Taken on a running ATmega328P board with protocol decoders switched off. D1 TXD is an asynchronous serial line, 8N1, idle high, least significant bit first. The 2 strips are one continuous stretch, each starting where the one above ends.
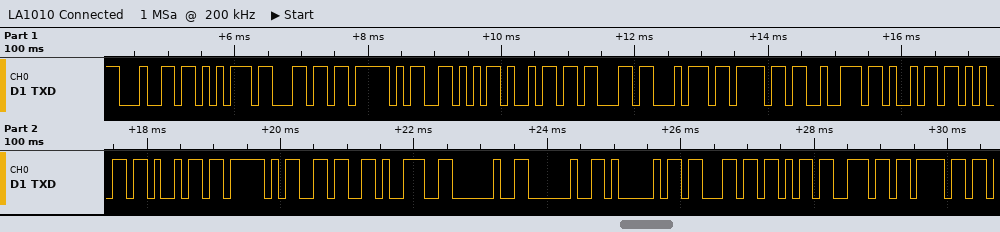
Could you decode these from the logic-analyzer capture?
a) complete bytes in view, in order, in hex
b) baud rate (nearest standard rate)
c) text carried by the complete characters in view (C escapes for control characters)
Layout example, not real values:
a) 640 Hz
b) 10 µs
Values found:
a) 64 75 6C 5F 56 69 63 74 6F 72 69 65 69 5F 36 39 20 20 41 63 6B 6E 6F
b) 9600 baud
c) "dul_Victoriei_69  Ackno"
